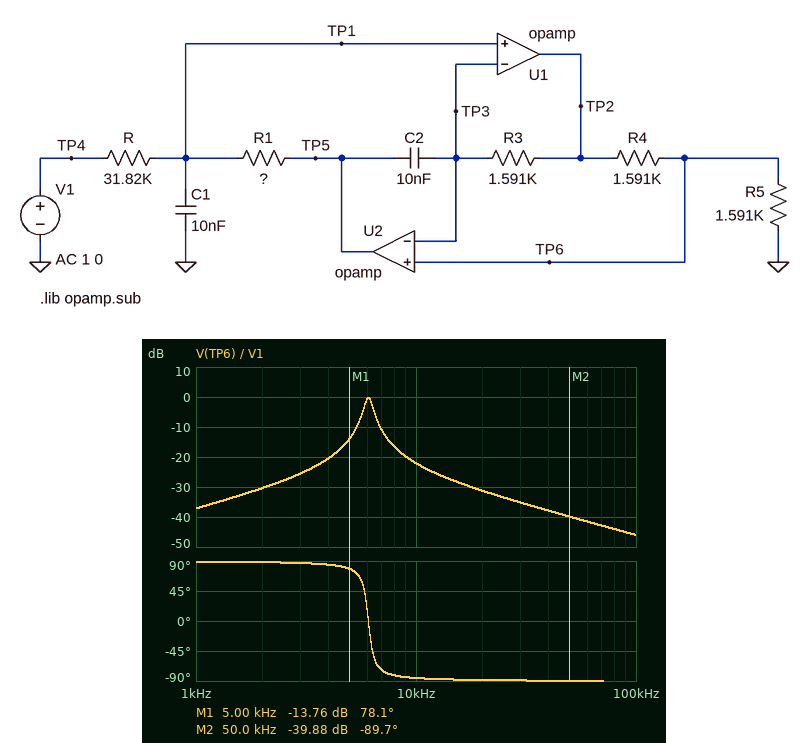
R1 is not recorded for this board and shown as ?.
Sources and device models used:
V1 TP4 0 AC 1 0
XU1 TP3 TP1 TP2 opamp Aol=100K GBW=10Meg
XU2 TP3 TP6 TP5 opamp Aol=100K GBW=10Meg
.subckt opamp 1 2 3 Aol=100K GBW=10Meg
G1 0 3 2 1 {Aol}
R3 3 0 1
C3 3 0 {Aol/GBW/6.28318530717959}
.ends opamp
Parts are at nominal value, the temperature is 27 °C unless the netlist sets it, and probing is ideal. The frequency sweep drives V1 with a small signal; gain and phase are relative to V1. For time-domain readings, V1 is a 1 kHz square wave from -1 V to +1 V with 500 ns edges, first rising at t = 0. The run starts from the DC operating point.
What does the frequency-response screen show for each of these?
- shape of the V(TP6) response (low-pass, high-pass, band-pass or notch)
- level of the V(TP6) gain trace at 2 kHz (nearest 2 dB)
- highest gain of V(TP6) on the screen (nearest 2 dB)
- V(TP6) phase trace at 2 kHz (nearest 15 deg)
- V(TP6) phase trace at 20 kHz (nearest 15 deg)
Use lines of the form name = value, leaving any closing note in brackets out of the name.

shape of the V(TP6) response = band-pass
level of the V(TP6) gain trace at 2 kHz = -30 dB
highest gain of V(TP6) on the screen = 0 dB
V(TP6) phase trace at 2 kHz = 90 deg
V(TP6) phase trace at 20 kHz = -90 deg
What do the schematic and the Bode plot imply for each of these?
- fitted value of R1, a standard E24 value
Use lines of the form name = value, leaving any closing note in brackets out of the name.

fitted value of R1, a standard E24 value = 4.3 kΩ
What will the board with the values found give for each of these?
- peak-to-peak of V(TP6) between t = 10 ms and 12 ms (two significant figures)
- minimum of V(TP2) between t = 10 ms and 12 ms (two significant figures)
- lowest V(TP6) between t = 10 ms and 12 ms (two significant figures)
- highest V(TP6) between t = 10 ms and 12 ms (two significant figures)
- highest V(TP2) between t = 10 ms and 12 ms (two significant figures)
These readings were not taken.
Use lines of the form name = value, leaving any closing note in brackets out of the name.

peak-to-peak of V(TP6) between t = 10 ms and 12 ms = 210 mV
minimum of V(TP2) between t = 10 ms and 12 ms = -210 mV
lowest V(TP6) between t = 10 ms and 12 ms = -110 mV
highest V(TP6) between t = 10 ms and 12 ms = 110 mV
highest V(TP2) between t = 10 ms and 12 ms = 210 mV
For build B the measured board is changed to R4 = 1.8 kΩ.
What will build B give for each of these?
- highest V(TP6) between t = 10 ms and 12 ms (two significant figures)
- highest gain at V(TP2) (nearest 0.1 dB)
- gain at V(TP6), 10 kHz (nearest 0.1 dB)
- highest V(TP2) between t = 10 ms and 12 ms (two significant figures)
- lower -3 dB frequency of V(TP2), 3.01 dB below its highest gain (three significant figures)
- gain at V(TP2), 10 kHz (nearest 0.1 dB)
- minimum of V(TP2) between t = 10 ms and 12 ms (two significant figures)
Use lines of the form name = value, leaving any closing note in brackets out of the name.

highest V(TP6) between t = 10 ms and 12 ms = 120 mV
highest gain at V(TP2) = 6.6 dB
gain at V(TP6), 10 kHz = -21.4 dB
highest V(TP2) between t = 10 ms and 12 ms = 260 mV
lower -3 dB frequency of V(TP2), 3.01 dB below its highest gain = 6.22 kHz
gain at V(TP2), 10 kHz = -14.8 dB
minimum of V(TP2) between t = 10 ms and 12 ms = -260 mV
